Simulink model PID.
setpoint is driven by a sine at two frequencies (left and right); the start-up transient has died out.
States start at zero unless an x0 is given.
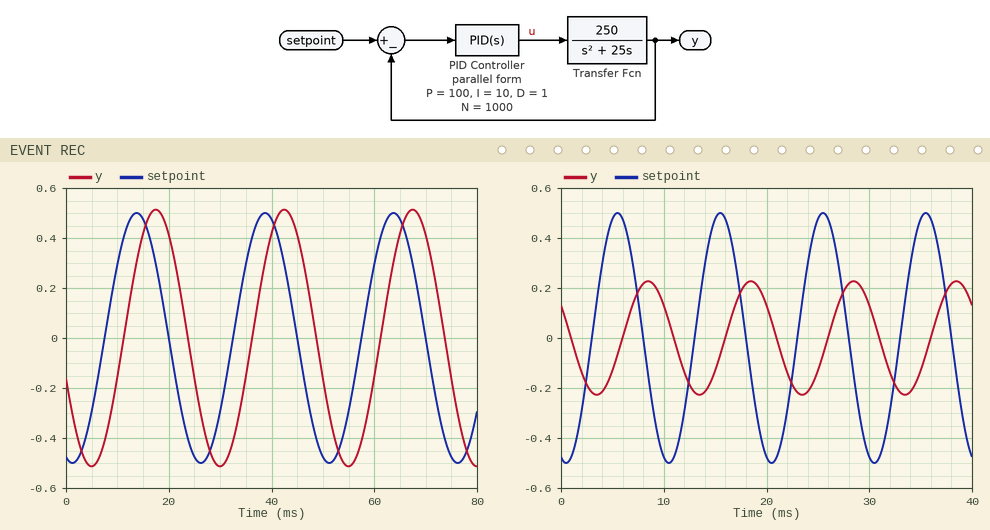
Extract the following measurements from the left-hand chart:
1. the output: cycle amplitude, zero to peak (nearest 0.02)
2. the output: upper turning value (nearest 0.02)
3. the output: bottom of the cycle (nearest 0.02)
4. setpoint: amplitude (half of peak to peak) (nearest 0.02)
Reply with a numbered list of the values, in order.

1. 0.52
2. 0.52
3. -0.52
4. 0.50
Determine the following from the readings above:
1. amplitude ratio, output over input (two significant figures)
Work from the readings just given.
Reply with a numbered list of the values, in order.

1. 1.0
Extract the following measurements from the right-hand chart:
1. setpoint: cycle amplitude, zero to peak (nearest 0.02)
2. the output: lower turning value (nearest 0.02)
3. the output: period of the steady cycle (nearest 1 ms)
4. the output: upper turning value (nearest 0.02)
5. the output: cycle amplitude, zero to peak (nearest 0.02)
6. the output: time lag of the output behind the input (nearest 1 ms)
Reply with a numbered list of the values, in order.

1. 0.50
2. -0.22
3. 10 ms
4. 0.22
5. 0.22
6. 3 ms
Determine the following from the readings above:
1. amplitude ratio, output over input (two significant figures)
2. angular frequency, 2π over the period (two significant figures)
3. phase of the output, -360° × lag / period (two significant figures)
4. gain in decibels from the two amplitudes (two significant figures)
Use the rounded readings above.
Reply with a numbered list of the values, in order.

1. 0.44
2. 0.63 rad/ms
3. -110°
4. -7.1 dB
